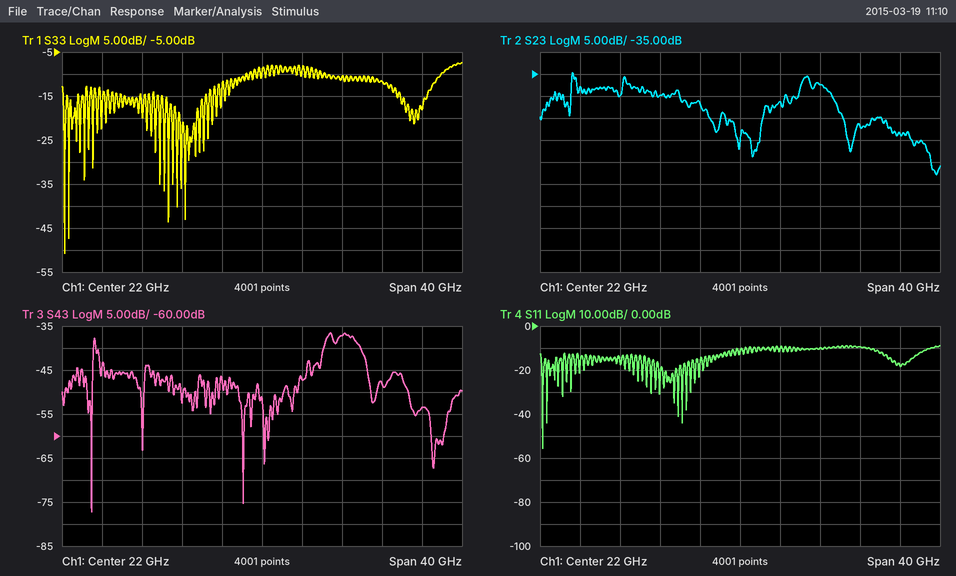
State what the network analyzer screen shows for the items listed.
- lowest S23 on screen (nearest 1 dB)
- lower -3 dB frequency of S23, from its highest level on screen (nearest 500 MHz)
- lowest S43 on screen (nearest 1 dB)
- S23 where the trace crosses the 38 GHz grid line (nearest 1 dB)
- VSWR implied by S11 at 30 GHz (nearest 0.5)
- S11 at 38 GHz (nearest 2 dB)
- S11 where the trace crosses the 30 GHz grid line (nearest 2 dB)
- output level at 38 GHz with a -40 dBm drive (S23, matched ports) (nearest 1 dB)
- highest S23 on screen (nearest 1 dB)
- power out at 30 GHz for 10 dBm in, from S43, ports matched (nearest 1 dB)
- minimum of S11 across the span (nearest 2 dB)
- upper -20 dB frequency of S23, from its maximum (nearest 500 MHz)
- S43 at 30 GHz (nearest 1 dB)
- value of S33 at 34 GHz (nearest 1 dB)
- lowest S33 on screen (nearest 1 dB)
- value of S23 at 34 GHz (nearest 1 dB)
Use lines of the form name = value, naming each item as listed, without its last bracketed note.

lowest S23 on screen = -58 dB
lower -3 dB frequency of S23, from its highest level on screen = 5.0 GHz
lowest S43 on screen = -77 dB
S23 where the trace crosses the 38 GHz grid line = -49 dB
VSWR implied by S11 at 30 GHz = 2.0
S11 at 38 GHz = -18 dB
S11 where the trace crosses the 30 GHz grid line = -10 dB
output level at 38 GHz with a -40 dBm drive (S23, matched ports) = -89 dBm
highest S23 on screen = -35 dB
power out at 30 GHz for 10 dBm in, from S43, ports matched = -27 dBm
minimum of S11 across the span = -56 dB
upper -20 dB frequency of S23, from its maximum = 41.0 GHz
S43 at 30 GHz = -37 dB
value of S33 at 34 GHz = -12 dB
lowest S33 on screen = -51 dB
value of S23 at 34 GHz = -47 dB
